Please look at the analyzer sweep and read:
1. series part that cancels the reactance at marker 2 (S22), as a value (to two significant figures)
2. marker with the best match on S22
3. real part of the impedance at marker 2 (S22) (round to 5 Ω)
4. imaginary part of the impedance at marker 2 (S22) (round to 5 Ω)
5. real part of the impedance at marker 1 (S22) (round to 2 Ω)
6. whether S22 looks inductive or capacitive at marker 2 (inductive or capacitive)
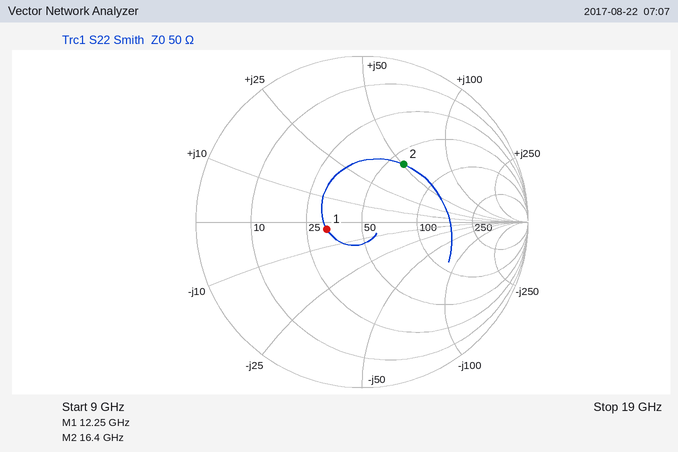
190 fF
marker 1
60 Ω
+50 Ω
32 Ω
inductive
